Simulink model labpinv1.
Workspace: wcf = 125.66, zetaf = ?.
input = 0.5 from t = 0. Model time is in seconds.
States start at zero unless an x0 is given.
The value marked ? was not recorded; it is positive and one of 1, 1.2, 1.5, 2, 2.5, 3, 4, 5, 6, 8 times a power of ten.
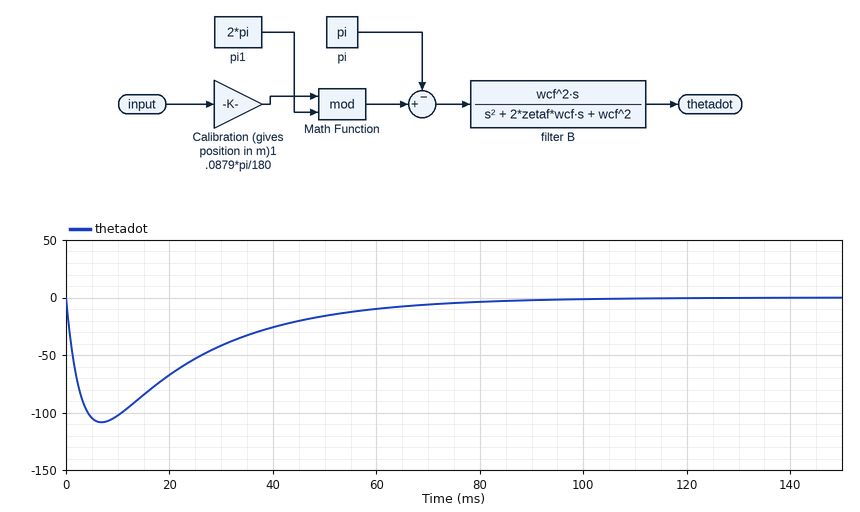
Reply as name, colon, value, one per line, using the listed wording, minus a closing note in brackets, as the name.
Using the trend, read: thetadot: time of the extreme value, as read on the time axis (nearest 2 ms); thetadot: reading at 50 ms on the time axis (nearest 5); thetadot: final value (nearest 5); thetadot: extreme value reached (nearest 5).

thetadot: time of the extreme value, as read on the time axis: 6 ms
thetadot: reading at 50 ms on the time axis: -15
thetadot: final value: 0
thetadot: extreme value reached: -110
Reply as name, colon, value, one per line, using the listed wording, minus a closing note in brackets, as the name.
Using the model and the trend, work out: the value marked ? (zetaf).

the value marked ?: 1.5
